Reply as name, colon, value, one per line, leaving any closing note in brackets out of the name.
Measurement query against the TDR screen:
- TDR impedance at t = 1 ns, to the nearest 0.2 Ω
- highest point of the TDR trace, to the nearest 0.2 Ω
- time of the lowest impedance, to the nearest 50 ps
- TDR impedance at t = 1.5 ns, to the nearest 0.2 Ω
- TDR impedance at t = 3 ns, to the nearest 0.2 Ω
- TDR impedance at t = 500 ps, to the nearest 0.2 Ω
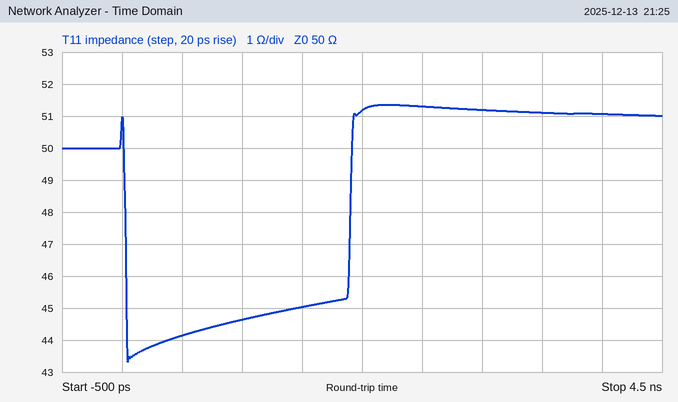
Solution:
TDR impedance at t = 1 ns, to the nearest 0.2 Ω: 44.6 Ω
highest point of the TDR trace, to the nearest 0.2 Ω: 51.4 Ω
time of the lowest impedance, to the nearest 50 ps: 50 ps
TDR impedance at t = 1.5 ns, to the nearest 0.2 Ω: 45.0 Ω
TDR impedance at t = 3 ns, to the nearest 0.2 Ω: 51.2 Ω
TDR impedance at t = 500 ps, to the nearest 0.2 Ω: 44.2 Ω
